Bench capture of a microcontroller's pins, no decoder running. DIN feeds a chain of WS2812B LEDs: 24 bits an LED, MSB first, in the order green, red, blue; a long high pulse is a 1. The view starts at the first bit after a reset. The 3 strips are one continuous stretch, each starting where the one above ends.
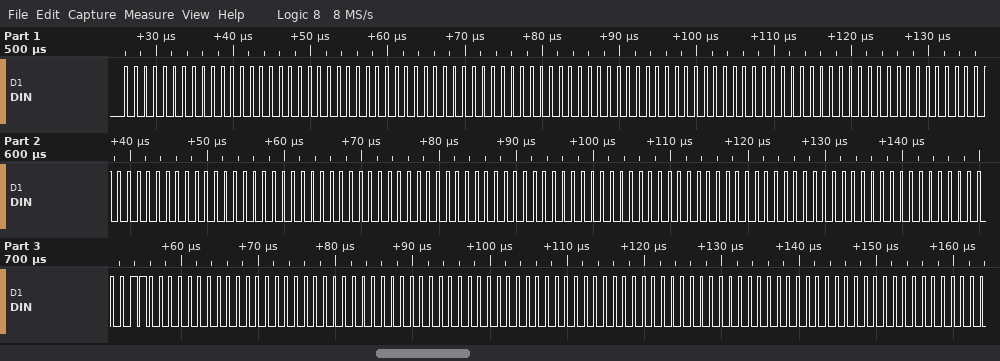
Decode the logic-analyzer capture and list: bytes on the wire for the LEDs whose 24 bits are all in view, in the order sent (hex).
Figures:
00 00 00 00 00 00 00 00 00 00 00 00 00 00 00 00 00 00 00 00 00 00 03 00 00 00 00 00 00 00 00 00 00
